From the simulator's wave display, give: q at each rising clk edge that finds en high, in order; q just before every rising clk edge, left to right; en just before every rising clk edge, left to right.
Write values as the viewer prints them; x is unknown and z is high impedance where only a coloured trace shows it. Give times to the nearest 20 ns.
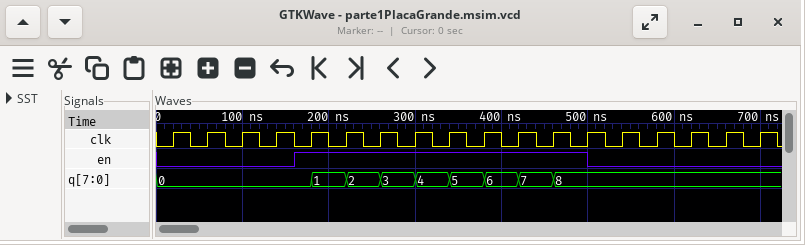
0, 1, 2, 3, 4, 5, 6, 7, 8
0, 0, 0, 0, 0, 1, 2, 3, 4, 5, 6, 7, 8, 8, 8, 8, 8, 8
0 0 0 0 1 1 1 1 1 1 1 1 1 0 0 0 0 0
